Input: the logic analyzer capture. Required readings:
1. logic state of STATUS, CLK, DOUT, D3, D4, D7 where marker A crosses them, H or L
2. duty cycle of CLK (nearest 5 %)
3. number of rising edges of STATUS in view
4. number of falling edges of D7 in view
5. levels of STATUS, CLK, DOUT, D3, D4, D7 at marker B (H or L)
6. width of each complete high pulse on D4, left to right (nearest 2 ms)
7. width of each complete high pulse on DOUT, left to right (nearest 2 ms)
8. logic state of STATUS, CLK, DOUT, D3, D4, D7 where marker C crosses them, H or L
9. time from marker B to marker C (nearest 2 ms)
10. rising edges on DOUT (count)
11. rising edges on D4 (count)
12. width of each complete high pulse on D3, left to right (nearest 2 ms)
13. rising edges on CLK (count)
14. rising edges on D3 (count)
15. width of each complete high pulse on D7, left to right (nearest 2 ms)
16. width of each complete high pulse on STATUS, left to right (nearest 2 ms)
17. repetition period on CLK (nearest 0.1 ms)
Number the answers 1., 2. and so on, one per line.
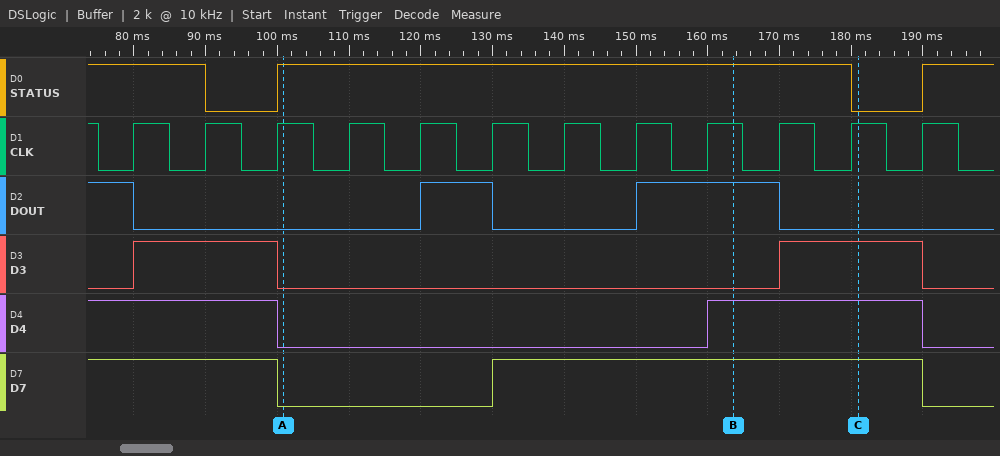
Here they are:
1. STATUS=H, CLK=H, DOUT=L, D3=L, D4=L, D7=L
2. 50 %
3. 2
4. 2
5. STATUS=H, CLK=H, DOUT=H, D3=L, D4=H, D7=H
6. 30 ms
7. 10 ms, 20 ms
8. STATUS=L, CLK=H, DOUT=L, D3=H, D4=H, D7=H
9. 18 ms
10. 2
11. 1
12. 20 ms, 20 ms
13. 12
14. 2
15. 60 ms
16. 80 ms
17. 10 ms
